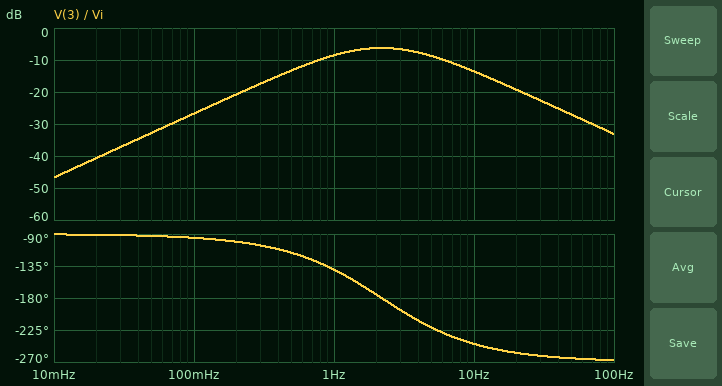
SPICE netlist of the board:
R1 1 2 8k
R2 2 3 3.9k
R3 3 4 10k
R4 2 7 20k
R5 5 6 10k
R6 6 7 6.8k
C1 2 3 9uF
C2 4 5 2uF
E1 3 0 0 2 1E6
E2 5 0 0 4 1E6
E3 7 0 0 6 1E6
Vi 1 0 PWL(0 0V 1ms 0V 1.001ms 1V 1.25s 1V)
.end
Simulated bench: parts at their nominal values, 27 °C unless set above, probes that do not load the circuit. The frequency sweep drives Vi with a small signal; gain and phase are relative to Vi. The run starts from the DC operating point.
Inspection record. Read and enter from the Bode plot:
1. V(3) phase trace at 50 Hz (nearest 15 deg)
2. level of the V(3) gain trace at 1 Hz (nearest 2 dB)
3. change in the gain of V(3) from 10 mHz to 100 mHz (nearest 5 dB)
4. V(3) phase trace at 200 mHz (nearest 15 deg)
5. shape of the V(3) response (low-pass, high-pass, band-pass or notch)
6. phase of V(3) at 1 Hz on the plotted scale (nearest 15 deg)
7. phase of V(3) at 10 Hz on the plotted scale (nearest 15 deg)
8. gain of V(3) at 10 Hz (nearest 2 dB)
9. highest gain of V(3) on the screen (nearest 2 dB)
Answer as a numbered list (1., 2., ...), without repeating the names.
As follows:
1. -270 deg
2. -8 dB
3. 20 dB
4. -105 deg
5. band-pass
6. -135 deg
7. -240 deg
8. -14 dB
9. -6 dB
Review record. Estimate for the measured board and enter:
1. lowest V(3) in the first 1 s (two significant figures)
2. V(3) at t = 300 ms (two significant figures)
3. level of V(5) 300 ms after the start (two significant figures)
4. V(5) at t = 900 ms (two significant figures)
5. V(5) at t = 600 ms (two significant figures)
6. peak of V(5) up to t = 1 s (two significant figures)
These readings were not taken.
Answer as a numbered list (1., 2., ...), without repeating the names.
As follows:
1. -360 mV
2. -72 mV
3. 3.3 V
4. 3.7 V
5. 3.7 V
6. 3.7 V
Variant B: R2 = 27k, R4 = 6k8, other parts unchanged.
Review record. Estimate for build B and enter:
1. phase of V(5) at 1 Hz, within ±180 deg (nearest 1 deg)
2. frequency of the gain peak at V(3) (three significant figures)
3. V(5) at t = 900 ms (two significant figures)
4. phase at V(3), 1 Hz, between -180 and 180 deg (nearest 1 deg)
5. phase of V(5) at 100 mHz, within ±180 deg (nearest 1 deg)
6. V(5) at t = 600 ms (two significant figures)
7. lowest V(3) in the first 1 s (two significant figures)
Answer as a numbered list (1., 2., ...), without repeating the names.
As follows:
1. -3 deg
2. 3.75 Hz
3. 1.4 V
4. -93 deg
5. 0 deg
6. 1.2 V
7. -520 mV
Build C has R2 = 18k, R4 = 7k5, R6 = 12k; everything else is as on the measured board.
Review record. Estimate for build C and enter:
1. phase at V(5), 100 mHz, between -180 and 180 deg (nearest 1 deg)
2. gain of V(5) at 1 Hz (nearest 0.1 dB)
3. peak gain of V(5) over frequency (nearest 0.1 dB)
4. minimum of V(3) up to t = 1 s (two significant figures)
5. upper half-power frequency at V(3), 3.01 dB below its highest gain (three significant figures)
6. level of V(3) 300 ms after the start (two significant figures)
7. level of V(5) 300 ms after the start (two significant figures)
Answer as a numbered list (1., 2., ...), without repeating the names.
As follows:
1. 0 deg
2. -1.8 dB
3. 11.6 dB
4. -400 mV
5. 5.26 Hz
6. -99 mV
7. 1.0 V
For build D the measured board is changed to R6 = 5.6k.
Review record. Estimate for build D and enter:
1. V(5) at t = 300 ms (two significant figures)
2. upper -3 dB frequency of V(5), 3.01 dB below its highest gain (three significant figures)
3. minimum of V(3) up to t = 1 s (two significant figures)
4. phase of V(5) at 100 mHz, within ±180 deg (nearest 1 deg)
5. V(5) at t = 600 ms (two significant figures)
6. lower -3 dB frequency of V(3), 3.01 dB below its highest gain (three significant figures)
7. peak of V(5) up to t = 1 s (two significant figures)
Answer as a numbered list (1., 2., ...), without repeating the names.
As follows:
1. 3.7 V
2. 1.06 Hz
3. -370 mV
4. -7 deg
5. 4.4 V
6. 746 mHz
7. 4.5 V
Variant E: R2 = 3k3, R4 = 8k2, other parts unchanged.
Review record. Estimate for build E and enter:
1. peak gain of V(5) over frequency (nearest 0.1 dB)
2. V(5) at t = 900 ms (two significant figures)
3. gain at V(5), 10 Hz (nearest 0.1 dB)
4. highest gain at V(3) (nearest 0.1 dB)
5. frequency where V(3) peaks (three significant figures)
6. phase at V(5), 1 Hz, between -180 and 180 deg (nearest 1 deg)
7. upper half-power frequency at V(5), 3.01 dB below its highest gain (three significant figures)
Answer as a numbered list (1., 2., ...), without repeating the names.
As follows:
1. 3.6 dB
2. 1.5 V
3. -15.4 dB
4. -7.7 dB
5. 3.42 Hz
6. -27 deg
7. 3.05 Hz
